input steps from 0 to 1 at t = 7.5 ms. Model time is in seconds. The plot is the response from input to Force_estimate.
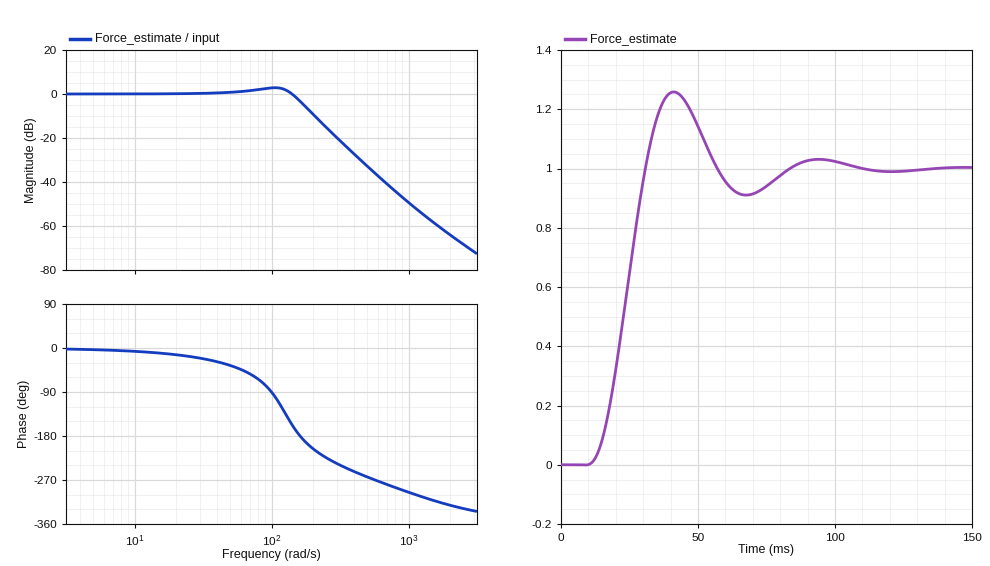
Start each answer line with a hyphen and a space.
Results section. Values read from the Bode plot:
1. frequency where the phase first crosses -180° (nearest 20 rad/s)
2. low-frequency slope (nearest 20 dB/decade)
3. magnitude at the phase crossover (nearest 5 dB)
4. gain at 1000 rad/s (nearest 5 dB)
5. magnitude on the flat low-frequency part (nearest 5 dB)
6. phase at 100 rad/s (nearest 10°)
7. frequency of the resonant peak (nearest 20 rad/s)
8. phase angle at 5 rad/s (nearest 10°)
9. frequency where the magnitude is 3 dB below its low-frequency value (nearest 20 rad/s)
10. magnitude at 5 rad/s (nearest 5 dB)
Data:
- 160 rad/s
- 0 dB/decade
- -5 dB
- -50 dB
- 0 dB
- -90°
- 100 rad/s
- 0°
- 160 rad/s
- 0 dB
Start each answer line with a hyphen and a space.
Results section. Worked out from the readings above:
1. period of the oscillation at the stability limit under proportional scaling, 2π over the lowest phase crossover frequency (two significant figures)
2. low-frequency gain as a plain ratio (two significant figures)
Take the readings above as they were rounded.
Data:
- 0.039 s
- 1.0
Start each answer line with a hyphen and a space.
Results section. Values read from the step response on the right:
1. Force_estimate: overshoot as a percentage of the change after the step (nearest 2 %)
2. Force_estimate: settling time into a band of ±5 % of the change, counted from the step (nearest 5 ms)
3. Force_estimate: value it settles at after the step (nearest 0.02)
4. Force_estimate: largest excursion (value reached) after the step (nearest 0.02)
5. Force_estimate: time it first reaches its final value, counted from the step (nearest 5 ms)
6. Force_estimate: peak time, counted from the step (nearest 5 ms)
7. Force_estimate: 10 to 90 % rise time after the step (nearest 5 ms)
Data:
- 26 %
- 70 ms
- 1.00
- 1.26
- 25 ms
- 35 ms
- 15 ms
